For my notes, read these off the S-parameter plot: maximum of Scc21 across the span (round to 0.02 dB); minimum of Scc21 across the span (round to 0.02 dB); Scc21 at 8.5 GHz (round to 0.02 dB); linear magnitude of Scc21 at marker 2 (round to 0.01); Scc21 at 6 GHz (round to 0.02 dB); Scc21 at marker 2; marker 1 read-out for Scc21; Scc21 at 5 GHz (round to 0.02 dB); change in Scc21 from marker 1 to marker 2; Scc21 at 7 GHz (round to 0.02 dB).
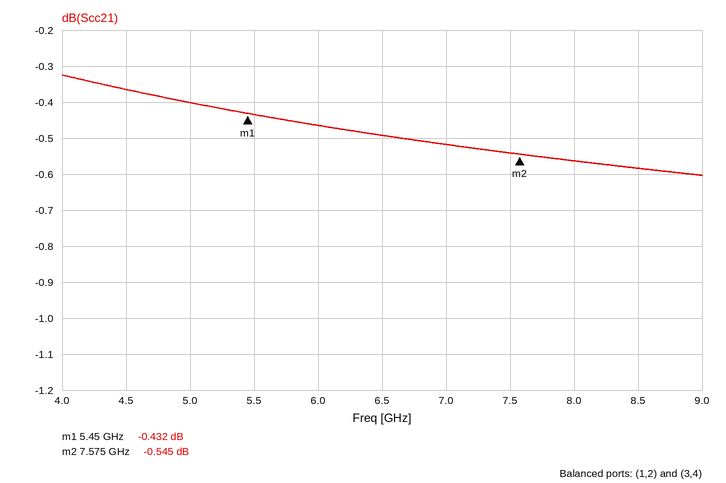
-0.32 dB
-0.60 dB
-0.58 dB
0.94
-0.46 dB
-0.545 dB
-0.432 dB
-0.40 dB
-0.113 dB
-0.52 dB
